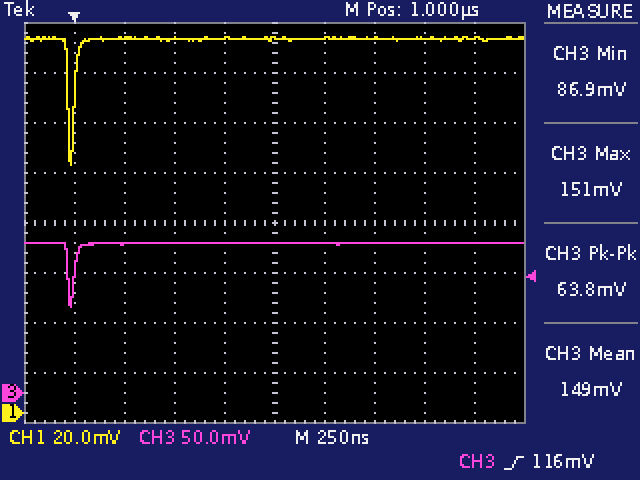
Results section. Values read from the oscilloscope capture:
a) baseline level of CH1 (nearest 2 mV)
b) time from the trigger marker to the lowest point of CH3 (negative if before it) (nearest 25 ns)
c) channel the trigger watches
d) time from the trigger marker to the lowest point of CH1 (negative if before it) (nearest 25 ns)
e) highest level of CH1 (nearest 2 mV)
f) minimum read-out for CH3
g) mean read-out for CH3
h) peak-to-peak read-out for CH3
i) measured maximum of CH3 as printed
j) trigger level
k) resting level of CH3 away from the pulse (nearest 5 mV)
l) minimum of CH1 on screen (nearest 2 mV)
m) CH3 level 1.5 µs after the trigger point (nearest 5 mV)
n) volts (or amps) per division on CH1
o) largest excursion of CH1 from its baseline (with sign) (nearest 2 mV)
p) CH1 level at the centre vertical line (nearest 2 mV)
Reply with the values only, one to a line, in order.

150 mV
-25 ns
CH3
-25 ns
150 mV
86.9 mV
149 mV
63.8 mV
151 mV
116 mV
150 mV
100 mV
150 mV
20 mV
-50 mV
150 mV
